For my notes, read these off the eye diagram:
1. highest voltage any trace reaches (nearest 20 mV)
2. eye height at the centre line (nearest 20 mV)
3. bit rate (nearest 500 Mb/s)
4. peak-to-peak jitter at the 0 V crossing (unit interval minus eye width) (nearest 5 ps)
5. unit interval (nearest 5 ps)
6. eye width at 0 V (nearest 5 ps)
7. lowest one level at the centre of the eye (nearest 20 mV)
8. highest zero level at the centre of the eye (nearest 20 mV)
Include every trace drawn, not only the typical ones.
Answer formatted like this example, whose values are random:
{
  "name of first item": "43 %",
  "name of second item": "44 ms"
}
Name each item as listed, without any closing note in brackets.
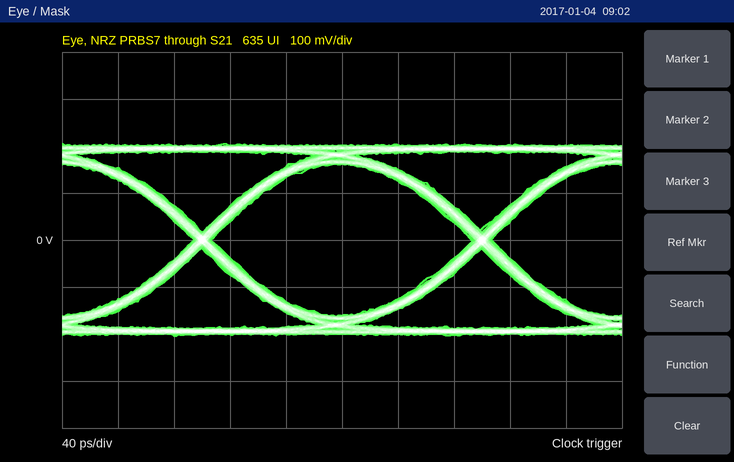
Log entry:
{
  "highest voltage any trace reaches": "200 mV",
  "eye height at the centre line": "320 mV",
  "bit rate": "5.0 Gb/s",
  "peak-to-peak jitter at the 0 V crossing (unit interval minus eye width)": "15 ps",
  "unit interval": "200 ps",
  "eye width at 0 V": "185 ps",
  "lowest one level at the centre of the eye": "160 mV",
  "highest zero level at the centre of the eye": "-160 mV"
}
